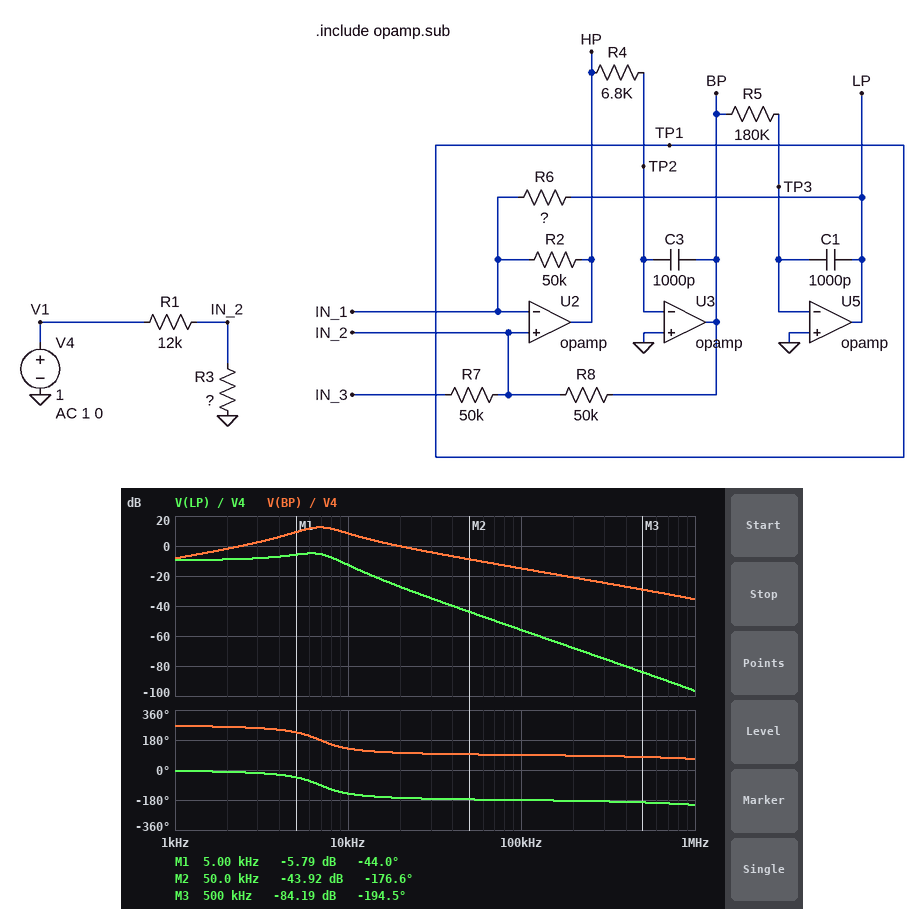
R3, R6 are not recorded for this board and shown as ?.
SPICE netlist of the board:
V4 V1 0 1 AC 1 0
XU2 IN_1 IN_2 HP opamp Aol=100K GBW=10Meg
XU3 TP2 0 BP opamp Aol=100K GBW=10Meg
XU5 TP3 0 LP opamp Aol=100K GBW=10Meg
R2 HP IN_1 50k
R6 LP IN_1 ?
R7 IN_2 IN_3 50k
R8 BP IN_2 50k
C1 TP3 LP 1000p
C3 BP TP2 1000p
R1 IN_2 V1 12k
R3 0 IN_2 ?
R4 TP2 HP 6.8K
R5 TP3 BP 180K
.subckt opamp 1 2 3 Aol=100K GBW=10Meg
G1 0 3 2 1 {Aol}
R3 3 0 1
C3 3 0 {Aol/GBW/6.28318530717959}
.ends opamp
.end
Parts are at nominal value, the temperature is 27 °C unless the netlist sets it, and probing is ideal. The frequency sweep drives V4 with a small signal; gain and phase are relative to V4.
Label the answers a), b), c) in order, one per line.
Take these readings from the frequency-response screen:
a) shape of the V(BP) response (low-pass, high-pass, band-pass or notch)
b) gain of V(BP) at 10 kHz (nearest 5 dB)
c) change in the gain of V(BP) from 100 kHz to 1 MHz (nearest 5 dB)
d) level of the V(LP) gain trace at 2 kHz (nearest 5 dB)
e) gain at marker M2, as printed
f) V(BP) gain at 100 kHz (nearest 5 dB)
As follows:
a) band-pass
b) 10 dB
c) -20 dB
d) -10 dB
e) -43.92 dB
f) -15 dB
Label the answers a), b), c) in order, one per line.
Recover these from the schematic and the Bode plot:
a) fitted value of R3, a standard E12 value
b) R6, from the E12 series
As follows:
a) 3.9 kΩ
b) 22 kΩ
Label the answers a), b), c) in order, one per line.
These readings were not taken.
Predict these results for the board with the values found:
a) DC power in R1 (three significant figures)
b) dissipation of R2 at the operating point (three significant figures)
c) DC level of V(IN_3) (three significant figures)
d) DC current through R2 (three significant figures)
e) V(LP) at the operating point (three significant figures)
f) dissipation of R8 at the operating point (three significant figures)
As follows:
a) 49.2 µW
b) 1.07 µW
c) 232 mV
d) 4.63 µA
e) 334 mV
f) 1.07 µW
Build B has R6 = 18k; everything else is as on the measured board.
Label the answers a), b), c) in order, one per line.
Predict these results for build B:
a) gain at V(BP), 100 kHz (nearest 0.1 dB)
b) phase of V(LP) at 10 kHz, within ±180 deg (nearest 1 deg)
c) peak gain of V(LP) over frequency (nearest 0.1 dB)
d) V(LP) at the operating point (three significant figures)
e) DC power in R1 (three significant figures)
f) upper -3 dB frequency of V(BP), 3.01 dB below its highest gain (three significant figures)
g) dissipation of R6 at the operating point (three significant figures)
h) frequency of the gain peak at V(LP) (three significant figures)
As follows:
a) -13.7 dB
b) -131 deg
c) -5.7 dB
d) 315 mV
e) 49.2 µW
f) 10.4 kHz
g) 386 nW
h) 6.75 kHz
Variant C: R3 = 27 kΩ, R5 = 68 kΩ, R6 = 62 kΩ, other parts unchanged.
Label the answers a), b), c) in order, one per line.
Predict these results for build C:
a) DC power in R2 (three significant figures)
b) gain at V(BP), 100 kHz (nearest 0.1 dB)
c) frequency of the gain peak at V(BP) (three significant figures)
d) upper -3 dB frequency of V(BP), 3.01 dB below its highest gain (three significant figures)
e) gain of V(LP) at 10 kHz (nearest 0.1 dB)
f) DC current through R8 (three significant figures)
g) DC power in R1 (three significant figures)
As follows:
a) 7.05 µW
b) -12.0 dB
c) 6.64 kHz
d) 10.3 kHz
e) -2.9 dB
f) 11.9 µA
g) 13.8 µW
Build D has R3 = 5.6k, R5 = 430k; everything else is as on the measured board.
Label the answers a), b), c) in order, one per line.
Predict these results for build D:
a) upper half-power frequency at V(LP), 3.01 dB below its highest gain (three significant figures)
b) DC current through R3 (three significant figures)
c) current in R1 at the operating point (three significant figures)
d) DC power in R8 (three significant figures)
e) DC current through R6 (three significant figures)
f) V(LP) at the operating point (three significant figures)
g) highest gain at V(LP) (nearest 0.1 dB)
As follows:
a) 4.90 kHz
b) 52.8 µA
c) 58.7 µA
d) 1.75 µW
e) 5.91 µA
f) 426 mV
g) -7.1 dB
